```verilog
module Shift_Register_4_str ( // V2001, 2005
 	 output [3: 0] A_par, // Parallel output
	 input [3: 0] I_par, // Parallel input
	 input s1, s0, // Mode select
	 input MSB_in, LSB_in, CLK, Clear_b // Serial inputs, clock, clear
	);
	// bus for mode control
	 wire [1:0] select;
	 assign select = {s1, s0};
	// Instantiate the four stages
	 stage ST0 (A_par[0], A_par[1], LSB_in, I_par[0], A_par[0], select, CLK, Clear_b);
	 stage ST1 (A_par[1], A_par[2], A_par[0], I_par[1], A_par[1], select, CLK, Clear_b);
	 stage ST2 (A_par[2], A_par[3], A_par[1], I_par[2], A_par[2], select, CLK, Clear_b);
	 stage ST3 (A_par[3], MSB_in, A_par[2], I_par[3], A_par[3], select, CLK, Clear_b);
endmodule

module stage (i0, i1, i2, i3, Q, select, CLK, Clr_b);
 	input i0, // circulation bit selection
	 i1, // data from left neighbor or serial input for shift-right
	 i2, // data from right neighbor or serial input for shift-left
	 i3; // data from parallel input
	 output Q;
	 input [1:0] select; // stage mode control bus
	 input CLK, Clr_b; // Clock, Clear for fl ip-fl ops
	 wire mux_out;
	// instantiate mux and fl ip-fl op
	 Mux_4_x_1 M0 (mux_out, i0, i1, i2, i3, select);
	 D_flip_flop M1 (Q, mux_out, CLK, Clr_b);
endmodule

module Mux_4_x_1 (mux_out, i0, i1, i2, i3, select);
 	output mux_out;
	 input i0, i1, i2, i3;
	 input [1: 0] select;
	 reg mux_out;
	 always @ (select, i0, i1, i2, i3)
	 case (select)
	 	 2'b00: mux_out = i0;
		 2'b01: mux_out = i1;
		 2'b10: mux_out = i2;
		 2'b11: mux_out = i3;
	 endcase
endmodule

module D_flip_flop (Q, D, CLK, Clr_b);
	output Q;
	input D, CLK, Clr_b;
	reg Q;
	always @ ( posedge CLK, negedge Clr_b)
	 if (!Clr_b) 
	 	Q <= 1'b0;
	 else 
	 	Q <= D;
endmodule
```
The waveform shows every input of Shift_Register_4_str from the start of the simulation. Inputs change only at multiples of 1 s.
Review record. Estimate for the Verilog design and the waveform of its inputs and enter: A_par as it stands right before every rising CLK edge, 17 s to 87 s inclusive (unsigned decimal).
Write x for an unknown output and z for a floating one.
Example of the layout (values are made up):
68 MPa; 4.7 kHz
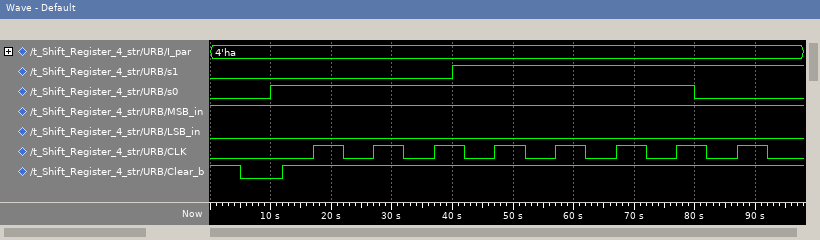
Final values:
0, 8, 12, 14, 10, 10, 10, 10
